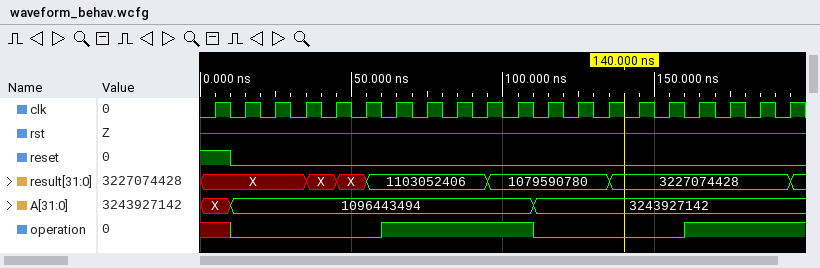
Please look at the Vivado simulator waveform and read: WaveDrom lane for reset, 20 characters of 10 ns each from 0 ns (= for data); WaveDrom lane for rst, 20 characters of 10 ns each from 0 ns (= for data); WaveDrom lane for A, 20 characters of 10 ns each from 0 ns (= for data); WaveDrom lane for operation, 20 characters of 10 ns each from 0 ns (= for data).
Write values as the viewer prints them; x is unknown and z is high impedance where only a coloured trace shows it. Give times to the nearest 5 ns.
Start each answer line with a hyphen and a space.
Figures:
- {name: 'reset', wave: '10..................'}
- {name: 'rst', wave: 'z...................'}
- {name: 'A', wave: 'x=.........=........', data: '1096443494 3243927142'}
- {name: 'operation', wave: 'x0....1....0....1...'}
